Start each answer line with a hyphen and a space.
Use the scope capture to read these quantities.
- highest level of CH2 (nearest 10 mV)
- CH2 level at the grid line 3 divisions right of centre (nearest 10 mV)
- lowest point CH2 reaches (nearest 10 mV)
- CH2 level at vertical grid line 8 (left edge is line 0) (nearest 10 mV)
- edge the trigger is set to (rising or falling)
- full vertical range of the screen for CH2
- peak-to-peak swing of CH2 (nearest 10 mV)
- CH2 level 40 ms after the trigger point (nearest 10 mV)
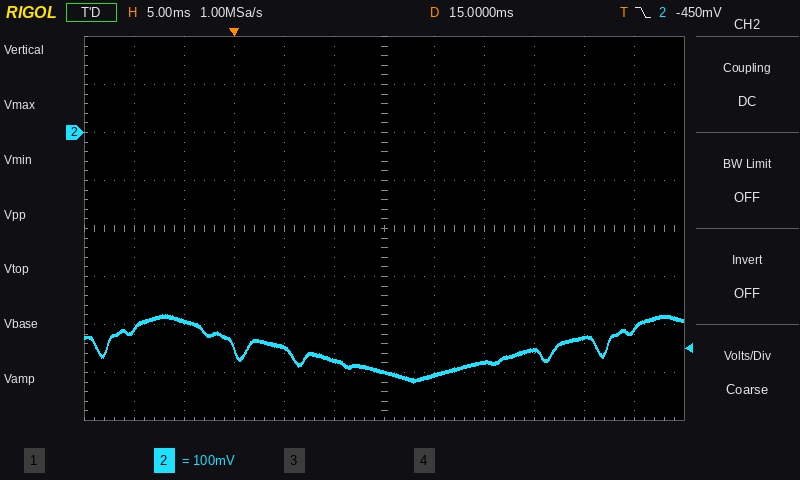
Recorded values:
- -380 mV
- -450 mV
- -520 mV
- -480 mV
- falling
- 800 mV
- 140 mV
- -410 mV
